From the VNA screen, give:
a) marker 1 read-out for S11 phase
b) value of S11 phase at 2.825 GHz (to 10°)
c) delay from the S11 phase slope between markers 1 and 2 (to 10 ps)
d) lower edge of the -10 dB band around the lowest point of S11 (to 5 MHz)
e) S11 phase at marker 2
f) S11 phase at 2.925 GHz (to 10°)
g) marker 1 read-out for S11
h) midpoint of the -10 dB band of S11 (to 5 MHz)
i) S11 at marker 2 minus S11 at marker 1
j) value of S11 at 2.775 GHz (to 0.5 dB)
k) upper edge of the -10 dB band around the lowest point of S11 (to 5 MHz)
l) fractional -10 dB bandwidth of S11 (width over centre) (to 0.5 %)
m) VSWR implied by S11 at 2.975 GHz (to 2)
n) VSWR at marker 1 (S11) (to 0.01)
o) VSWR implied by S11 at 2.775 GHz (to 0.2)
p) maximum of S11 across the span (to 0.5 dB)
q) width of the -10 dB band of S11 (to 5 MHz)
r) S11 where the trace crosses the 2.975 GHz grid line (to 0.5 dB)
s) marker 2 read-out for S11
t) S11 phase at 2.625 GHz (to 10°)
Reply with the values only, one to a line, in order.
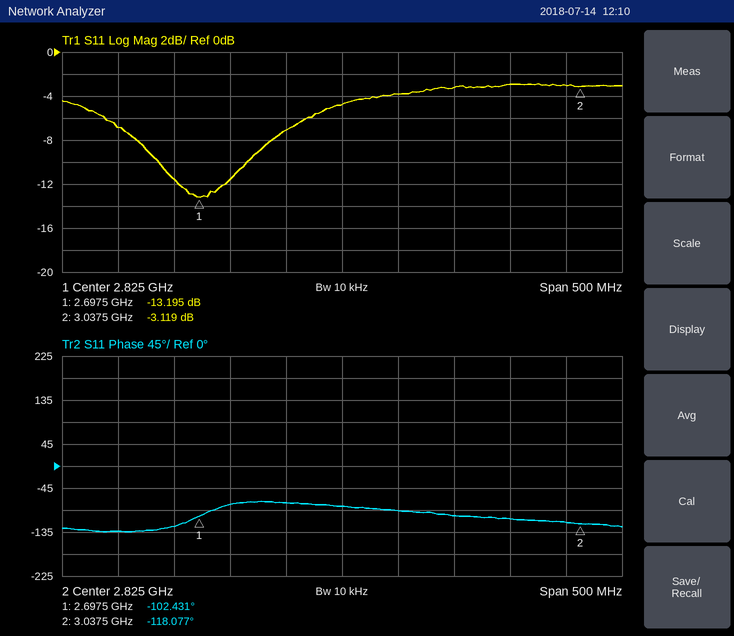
-102.431°
-80°
130 ps
2.660 GHz
-118.077°
-100°
-13.195 dB
2.700 GHz
10.076 dB
-7.0 dB
2.740 GHz
3.0 %
6
1.56
2.6
-3.0 dB
80 MHz
-3.0 dB
-3.119 dB
-130°
